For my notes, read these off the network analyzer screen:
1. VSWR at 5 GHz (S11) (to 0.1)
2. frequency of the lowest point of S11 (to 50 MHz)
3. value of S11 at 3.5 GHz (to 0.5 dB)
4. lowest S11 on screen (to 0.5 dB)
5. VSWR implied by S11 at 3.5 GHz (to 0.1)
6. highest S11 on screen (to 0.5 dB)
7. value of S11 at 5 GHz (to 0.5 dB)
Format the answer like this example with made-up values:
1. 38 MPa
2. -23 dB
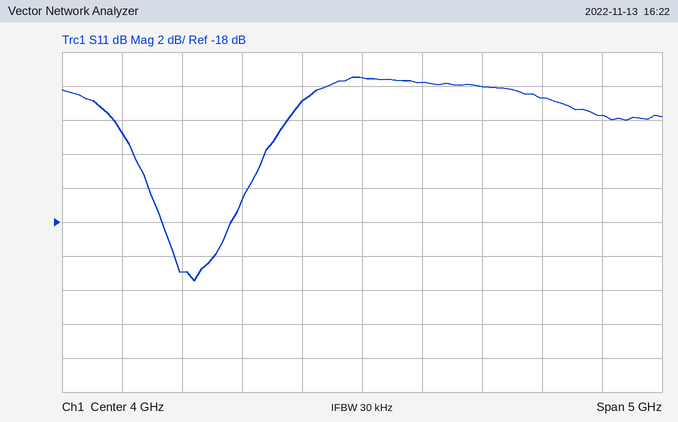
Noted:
1. 1.9
2. 2.60 GHz
3. -11.0 dB
4. -21.5 dB
5. 1.8
6. -9.5 dB
7. -10.0 dB
